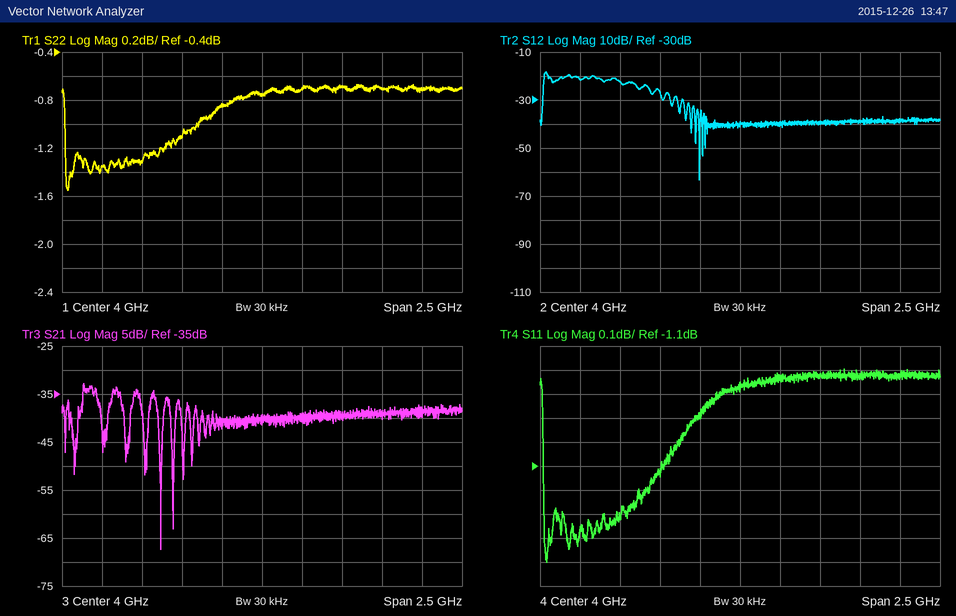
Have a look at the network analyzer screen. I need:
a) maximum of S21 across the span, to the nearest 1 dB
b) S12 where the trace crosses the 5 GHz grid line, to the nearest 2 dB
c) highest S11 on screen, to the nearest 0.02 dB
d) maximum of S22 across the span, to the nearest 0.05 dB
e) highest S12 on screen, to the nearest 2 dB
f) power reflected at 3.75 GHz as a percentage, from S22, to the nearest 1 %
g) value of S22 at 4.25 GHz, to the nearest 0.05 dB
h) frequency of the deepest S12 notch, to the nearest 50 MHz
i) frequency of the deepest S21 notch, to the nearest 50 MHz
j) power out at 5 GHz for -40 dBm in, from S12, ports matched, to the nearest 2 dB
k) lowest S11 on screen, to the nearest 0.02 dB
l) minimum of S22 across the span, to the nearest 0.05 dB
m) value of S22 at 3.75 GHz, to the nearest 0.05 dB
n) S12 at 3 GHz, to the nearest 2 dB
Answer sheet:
-33 dB
-38 dB
-0.70 dB
-0.65 dB
-18 dB
82 %
-0.70 dB
3.75 GHz
3.35 GHz
-78 dBm
-1.50 dB
-1.55 dB
-0.85 dB
-22 dB
